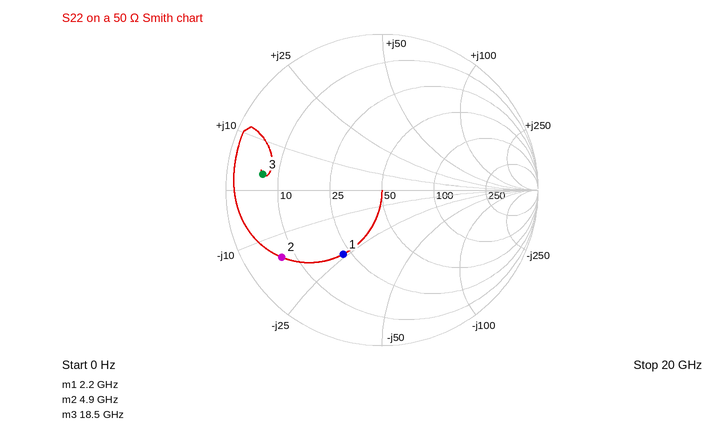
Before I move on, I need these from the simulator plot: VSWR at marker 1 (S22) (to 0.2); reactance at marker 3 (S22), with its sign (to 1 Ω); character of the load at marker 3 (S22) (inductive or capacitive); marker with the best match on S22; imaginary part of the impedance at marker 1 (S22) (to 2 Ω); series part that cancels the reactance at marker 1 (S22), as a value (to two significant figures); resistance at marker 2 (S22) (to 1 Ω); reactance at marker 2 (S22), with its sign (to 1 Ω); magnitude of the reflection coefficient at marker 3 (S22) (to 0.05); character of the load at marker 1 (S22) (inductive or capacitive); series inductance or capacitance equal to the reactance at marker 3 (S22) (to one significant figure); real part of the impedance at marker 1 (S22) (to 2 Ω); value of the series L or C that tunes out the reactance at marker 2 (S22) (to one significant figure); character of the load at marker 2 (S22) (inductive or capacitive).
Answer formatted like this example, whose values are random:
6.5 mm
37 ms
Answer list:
2.8
+3 Ω
inductive
marker 1
-24 Ω
1.7 nH
7 Ω
-15 Ω
0.75
capacitive
30 pH
22 Ω
500 pH
capacitive
